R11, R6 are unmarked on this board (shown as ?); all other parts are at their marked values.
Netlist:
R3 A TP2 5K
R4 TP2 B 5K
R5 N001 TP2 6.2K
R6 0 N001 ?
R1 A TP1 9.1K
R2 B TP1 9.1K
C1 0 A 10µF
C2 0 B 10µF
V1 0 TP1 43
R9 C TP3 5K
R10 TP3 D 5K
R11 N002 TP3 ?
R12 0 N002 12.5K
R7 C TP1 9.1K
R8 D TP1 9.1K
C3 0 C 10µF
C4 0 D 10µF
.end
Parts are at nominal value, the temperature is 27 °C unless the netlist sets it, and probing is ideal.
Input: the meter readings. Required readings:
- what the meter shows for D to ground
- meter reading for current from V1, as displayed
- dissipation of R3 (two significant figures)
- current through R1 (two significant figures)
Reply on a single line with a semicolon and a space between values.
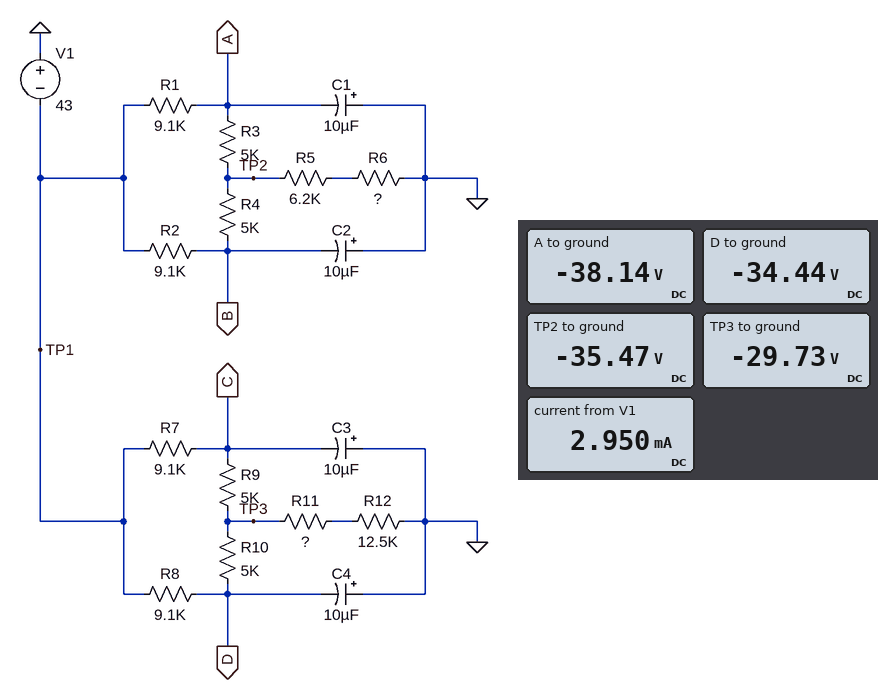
-34.44 V; 2.950 mA; 1.4 mW; 530 µA
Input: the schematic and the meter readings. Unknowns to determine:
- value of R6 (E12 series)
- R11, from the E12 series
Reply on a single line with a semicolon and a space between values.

27 kΩ; 3.3 kΩ
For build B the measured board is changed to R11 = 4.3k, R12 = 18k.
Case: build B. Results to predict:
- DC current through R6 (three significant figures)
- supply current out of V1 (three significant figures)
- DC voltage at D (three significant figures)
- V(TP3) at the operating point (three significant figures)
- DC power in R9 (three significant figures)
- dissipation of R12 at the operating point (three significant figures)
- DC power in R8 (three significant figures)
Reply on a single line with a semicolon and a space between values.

1.07 mA; 2.53 mA; -36.3 V; -32.7 V; 2.68 mW; 38.6 mW; 4.88 mW
